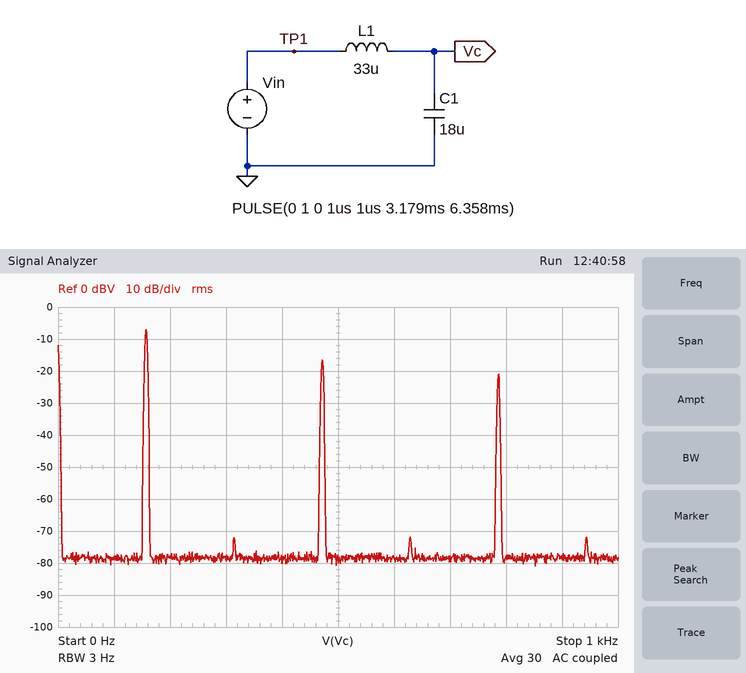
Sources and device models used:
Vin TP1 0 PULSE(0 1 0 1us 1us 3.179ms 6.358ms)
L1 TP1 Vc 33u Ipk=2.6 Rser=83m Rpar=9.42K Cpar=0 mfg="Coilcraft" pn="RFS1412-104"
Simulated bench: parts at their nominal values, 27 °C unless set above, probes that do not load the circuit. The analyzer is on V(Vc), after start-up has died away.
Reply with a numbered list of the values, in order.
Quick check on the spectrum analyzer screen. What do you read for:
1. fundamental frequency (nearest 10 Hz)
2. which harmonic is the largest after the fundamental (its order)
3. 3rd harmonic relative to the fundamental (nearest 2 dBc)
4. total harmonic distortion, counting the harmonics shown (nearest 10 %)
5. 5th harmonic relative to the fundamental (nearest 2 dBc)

1. 160 Hz
2. 3
3. -10 dBc
4. 40 %
5. -14 dBc
